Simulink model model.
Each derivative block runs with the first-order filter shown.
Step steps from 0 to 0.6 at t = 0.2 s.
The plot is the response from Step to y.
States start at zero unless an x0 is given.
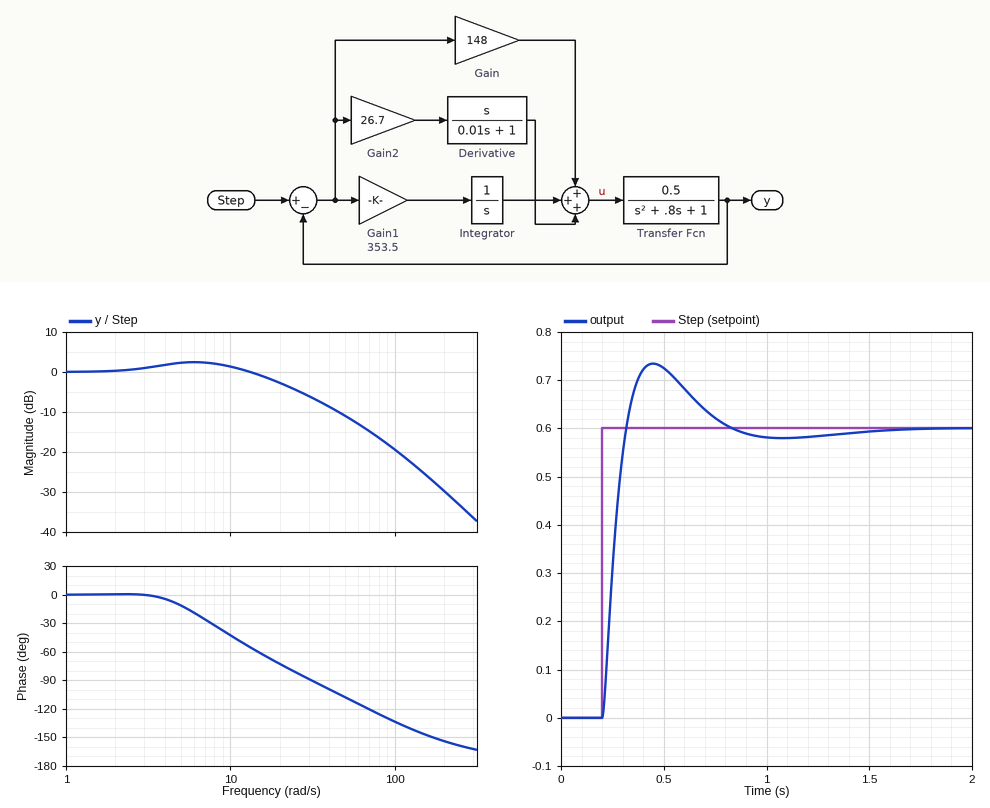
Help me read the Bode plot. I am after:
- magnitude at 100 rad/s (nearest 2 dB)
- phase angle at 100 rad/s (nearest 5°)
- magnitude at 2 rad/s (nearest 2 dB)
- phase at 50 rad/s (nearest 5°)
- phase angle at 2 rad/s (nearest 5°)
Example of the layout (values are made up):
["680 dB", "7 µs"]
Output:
["-20 dB", "-135°", "0 dB", "-110°", "0°"]
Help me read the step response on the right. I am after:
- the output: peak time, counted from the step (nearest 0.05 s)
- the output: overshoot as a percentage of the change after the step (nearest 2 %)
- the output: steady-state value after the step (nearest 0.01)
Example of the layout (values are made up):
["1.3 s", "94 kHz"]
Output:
["0.25 s", "22 %", "0.60"]
